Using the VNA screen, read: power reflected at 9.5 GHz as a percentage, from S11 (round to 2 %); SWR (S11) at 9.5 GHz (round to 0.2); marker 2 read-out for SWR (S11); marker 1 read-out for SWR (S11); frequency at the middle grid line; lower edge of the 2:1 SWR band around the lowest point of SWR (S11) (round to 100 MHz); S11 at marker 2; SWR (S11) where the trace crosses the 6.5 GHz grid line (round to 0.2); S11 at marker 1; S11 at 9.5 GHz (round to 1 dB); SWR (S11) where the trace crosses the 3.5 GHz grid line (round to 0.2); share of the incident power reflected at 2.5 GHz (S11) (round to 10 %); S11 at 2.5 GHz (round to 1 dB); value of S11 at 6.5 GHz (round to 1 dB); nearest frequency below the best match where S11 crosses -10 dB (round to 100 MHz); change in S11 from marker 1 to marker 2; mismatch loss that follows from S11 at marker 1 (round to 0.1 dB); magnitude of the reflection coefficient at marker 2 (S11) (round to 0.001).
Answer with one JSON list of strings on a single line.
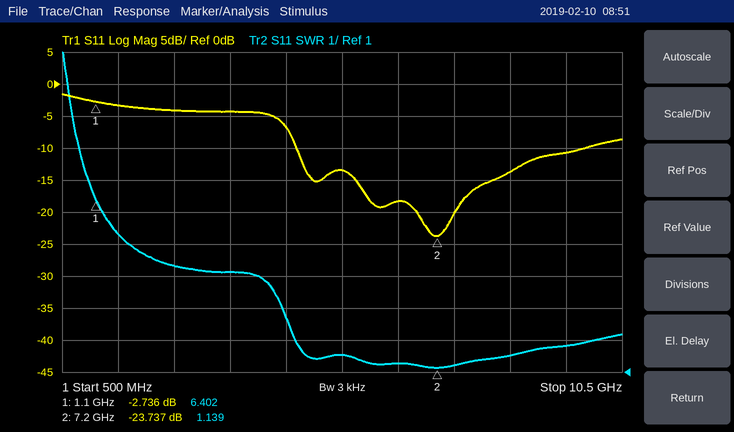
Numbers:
["8 %", "1.8", "1.139", "6.402", "5.5 GHz", "4.7 GHz", "-23.737 dB", "1.2", "-2.736 dB", "-11 dB", "4.2", "40 %", "-4 dB", "-18 dB", "4.7 GHz", "-21.001 dB", "3.3 dB", "0.065"]
